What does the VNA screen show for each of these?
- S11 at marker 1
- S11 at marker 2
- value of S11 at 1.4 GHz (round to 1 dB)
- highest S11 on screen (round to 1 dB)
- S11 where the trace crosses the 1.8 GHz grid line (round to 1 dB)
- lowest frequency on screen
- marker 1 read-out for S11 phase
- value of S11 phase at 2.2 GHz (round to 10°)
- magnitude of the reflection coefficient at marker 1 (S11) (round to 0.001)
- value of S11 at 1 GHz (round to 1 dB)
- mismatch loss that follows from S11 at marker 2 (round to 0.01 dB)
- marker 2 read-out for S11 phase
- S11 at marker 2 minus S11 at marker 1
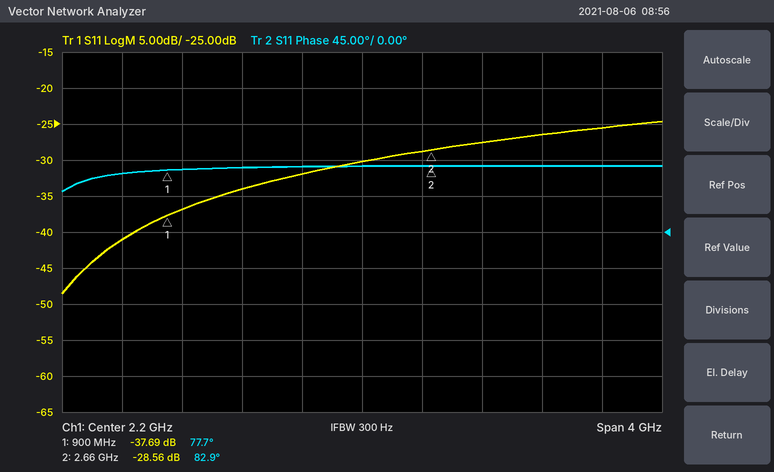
-37.69 dB
-28.56 dB
-34 dB
-25 dB
-32 dB
200 MHz
77.7°
80°
0.013
-37 dB
0.01 dB
82.9°
9.13 dB
